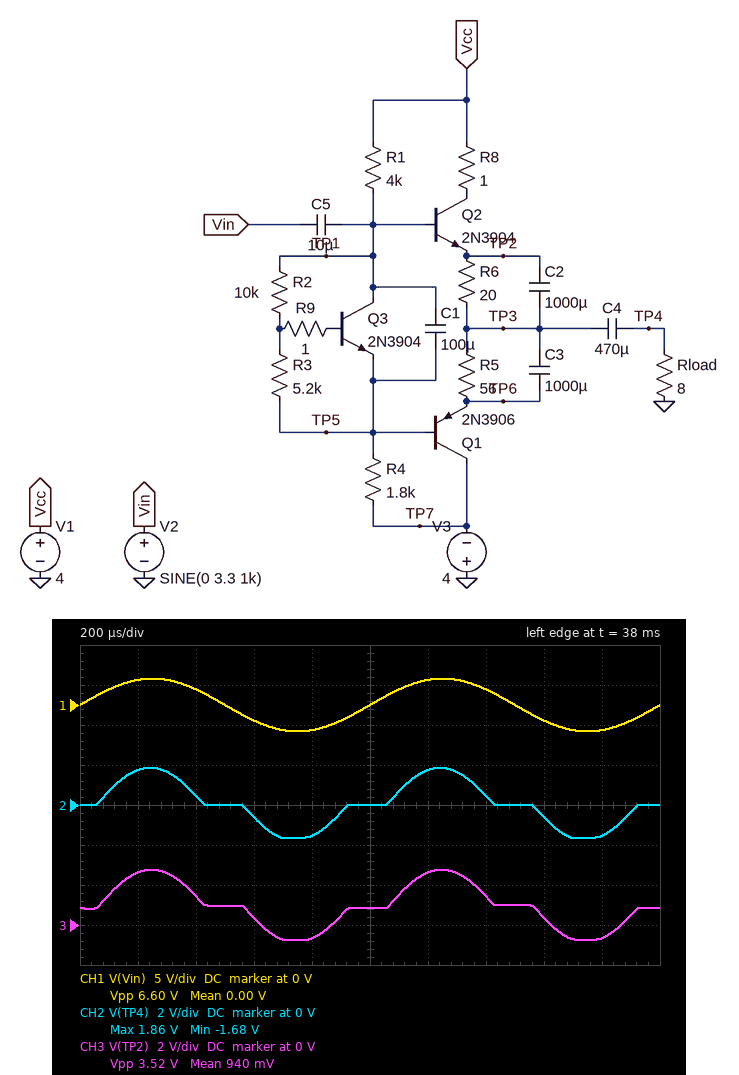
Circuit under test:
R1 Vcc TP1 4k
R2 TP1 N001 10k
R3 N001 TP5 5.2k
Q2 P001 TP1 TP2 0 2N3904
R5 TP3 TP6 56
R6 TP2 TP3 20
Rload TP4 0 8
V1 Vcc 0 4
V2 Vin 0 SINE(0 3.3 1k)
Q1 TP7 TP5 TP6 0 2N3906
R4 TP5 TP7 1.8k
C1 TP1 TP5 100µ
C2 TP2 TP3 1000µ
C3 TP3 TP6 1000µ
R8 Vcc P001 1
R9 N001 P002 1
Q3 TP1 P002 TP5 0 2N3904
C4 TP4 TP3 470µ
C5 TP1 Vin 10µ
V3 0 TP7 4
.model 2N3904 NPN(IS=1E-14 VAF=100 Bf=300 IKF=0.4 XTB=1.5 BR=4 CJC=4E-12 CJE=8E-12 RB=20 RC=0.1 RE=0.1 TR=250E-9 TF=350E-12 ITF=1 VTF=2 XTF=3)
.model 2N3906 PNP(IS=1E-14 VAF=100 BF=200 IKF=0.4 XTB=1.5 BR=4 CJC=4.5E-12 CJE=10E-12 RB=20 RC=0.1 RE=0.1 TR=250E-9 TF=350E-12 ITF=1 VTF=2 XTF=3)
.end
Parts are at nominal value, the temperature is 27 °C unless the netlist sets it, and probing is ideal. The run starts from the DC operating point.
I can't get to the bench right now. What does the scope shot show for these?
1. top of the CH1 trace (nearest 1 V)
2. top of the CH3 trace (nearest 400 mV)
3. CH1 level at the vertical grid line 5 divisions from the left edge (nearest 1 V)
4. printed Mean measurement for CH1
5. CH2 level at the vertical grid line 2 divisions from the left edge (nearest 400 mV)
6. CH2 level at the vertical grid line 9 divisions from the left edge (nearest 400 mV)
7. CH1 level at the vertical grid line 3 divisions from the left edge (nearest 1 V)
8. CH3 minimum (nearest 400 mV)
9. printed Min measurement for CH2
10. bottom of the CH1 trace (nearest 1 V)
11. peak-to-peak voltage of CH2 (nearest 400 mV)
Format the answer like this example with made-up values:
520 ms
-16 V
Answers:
3 V
2.8 V
0 V
0.00 V
400 mV
-1.6 V
-2 V
-800 mV
-1.68 V
-3 V
3.6 V
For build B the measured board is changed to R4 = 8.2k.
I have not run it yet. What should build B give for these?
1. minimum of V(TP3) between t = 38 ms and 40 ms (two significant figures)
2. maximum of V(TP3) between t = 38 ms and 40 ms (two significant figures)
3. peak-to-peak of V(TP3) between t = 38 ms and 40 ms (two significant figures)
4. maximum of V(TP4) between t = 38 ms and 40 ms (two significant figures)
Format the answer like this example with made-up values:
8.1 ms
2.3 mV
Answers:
-810 mV
2.6 V
3.4 V
1.7 V
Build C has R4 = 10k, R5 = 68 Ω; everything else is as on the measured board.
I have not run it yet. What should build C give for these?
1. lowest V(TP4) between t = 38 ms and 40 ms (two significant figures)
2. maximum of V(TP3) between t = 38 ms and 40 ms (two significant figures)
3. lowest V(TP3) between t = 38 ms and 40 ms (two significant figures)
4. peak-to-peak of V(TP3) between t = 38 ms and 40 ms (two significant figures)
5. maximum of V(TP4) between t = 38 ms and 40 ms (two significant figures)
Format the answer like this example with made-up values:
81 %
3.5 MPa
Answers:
-1.6 V
2.7 V
-630 mV
3.3 V
1.7 V
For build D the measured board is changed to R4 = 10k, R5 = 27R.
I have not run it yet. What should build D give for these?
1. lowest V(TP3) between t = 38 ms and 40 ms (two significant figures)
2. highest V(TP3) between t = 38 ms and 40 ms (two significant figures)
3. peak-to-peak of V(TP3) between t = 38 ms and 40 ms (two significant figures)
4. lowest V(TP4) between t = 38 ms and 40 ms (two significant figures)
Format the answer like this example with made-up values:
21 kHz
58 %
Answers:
-1.2 V
2.5 V
3.8 V
-1.9 V
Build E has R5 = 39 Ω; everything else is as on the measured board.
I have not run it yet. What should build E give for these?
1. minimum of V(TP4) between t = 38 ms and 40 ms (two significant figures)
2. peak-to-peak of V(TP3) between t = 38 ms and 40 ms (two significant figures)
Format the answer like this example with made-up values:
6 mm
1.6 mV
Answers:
-1.8 V
3.7 V
